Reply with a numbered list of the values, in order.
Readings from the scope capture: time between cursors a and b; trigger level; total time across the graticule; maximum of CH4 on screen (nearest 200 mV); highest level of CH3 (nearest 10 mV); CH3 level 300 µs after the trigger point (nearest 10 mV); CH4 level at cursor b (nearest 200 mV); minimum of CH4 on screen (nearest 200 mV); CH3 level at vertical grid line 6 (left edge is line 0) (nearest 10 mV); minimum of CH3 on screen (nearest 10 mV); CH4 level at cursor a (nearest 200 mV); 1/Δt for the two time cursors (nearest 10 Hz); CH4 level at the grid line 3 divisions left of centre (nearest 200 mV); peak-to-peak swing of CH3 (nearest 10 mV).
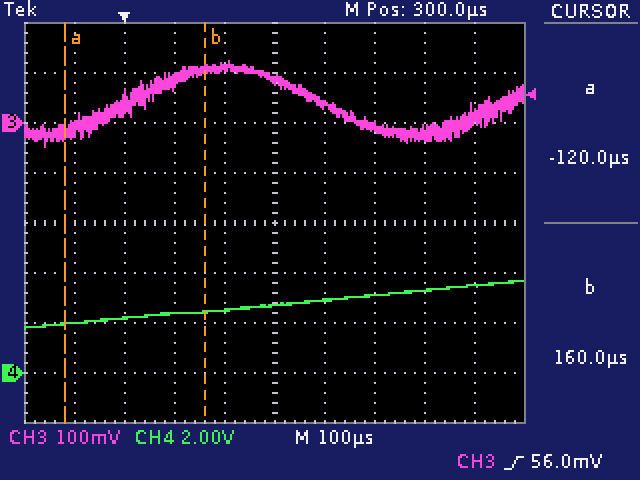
1. 280 µs
2. 56.0 mV
3. 1 ms
4. 3.6 V
5. 120 mV
6. 90 mV
7. 2.4 V
8. 1.8 V
9. 40 mV
10. -50 mV
11. 2.0 V
12. 3.57 kHz
13. 2.2 V
14. 170 mV
